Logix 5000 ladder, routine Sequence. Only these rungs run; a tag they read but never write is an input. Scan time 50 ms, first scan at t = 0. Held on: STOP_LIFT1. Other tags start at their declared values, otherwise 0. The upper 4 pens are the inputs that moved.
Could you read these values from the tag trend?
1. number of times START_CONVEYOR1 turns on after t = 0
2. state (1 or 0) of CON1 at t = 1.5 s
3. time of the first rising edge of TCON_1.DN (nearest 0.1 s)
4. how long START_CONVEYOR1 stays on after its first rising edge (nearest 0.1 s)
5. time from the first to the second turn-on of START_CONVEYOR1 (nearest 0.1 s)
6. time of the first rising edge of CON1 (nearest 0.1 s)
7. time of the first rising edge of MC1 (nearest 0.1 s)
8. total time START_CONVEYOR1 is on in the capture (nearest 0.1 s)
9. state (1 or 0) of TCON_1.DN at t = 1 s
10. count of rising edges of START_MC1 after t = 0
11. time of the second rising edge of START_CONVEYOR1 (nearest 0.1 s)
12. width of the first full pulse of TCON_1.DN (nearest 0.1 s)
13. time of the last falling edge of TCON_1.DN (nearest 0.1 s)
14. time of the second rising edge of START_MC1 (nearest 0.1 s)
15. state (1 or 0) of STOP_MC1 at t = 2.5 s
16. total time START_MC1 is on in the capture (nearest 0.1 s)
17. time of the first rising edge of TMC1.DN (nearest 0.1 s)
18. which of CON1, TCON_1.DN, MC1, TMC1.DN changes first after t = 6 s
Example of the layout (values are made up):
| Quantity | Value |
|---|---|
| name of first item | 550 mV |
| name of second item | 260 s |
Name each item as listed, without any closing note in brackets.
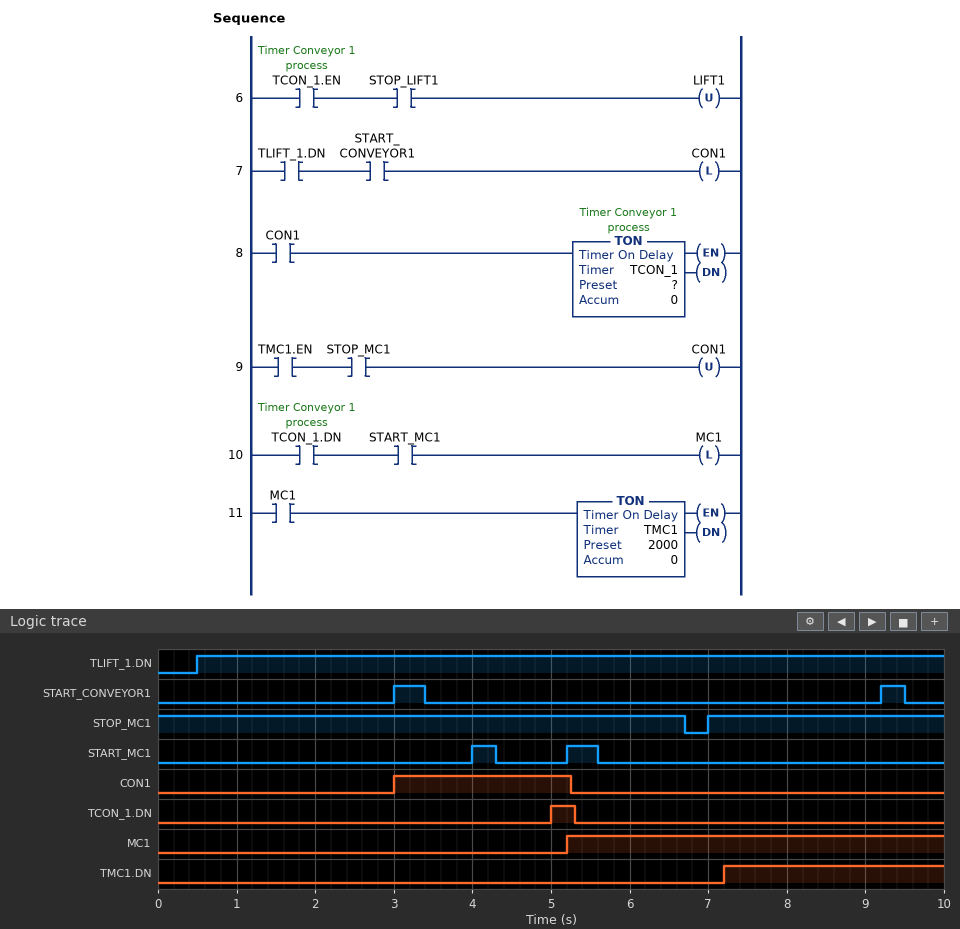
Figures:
| Quantity | Value |
|---|---|
| number of times START_CONVEYOR1 turns on after t = 0 | 2 |
| state (1 or 0) of CON1 at t = 1.5 s | 0 |
| time of the first rising edge of TCON_1.DN | 5.0 s |
| how long START_CONVEYOR1 stays on after its first rising edge | 0.4 s |
| time from the first to the second turn-on of START_CONVEYOR1 | 6.2 s |
| time of the first rising edge of CON1 | 3.0 s |
| time of the first rising edge of MC1 | 5.2 s |
| total time START_CONVEYOR1 is on in the capture | 0.7 s |
| state (1 or 0) of TCON_1.DN at t = 1 s | 0 |
| count of rising edges of START_MC1 after t = 0 | 2 |
| time of the second rising edge of START_CONVEYOR1 | 9.2 s |
| width of the first full pulse of TCON_1.DN | 0.3 s |
| time of the last falling edge of TCON_1.DN | 5.3 s |
| time of the second rising edge of START_MC1 | 5.2 s |
| state (1 or 0) of STOP_MC1 at t = 2.5 s | 1 |
| total time START_MC1 is on in the capture | 0.7 s |
| time of the first rising edge of TMC1.DN | 7.2 s |
| which of CON1, TCON_1.DN, MC1, TMC1.DN changes first after t = 6 s | TMC1.DN |
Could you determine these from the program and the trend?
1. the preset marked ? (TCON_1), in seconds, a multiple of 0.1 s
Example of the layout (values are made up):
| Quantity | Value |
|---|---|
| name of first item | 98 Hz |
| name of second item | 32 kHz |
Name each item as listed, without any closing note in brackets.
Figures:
| Quantity | Value |
|---|---|
| the preset marked ? (TCON_1), in seconds, a multiple of 0.1 s | 2.0 s |
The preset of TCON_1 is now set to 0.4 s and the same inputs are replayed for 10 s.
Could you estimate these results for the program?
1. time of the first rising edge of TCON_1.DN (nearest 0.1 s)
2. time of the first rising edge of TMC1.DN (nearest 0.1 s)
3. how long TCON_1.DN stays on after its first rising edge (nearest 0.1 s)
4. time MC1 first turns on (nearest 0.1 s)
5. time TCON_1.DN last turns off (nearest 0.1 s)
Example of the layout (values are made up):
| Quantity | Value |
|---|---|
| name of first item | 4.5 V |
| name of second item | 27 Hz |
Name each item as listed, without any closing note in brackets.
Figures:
| Quantity | Value |
|---|---|
| time of the first rising edge of TCON_1.DN | 3.4 s |
| time of the first rising edge of TMC1.DN | 6.0 s |
| how long TCON_1.DN stays on after its first rising edge | 0.7 s |
| time MC1 first turns on | 4.0 s |
| time TCON_1.DN last turns off | 4.1 s |
